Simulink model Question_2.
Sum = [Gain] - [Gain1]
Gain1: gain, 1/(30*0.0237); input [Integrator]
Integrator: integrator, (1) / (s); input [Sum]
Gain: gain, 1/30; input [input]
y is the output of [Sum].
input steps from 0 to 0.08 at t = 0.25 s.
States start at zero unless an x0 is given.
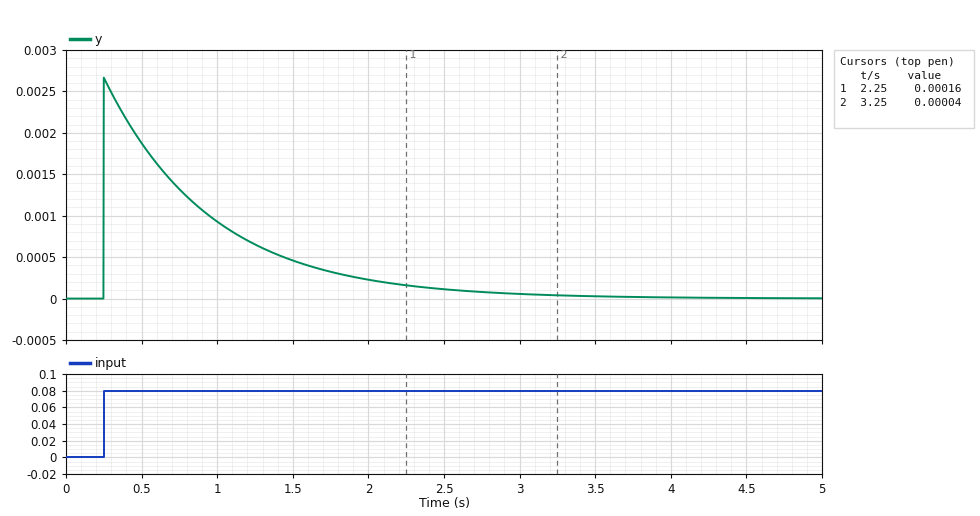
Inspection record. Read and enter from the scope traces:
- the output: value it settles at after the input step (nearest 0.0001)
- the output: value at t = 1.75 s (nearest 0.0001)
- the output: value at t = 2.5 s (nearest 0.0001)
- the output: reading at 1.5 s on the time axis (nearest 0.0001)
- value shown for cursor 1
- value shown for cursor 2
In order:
0.0000
0.0003
0.0001
0.0005
0.00016
0.00004
